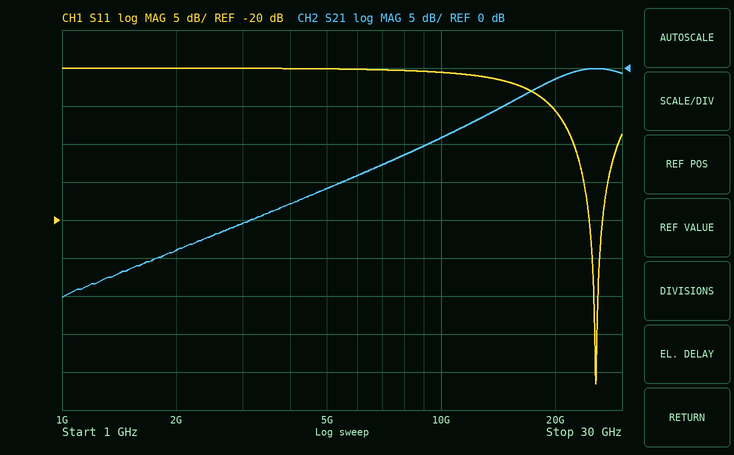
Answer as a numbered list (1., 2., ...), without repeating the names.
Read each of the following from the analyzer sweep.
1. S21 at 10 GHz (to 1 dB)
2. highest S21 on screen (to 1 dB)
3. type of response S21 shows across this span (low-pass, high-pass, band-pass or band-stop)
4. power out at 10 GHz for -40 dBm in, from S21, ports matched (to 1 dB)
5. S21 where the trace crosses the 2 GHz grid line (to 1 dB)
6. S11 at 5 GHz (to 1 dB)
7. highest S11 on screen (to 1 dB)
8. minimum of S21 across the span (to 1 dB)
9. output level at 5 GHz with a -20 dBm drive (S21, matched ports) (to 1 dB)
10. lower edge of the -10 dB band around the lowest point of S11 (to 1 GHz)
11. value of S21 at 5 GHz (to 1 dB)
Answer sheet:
1. -9 dB
2. 0 dB
3. high-pass
4. -49 dBm
5. -24 dB
6. 0 dB
7. 0 dB
8. -30 dB
9. -36 dBm
10. 22 GHz
11. -16 dB
